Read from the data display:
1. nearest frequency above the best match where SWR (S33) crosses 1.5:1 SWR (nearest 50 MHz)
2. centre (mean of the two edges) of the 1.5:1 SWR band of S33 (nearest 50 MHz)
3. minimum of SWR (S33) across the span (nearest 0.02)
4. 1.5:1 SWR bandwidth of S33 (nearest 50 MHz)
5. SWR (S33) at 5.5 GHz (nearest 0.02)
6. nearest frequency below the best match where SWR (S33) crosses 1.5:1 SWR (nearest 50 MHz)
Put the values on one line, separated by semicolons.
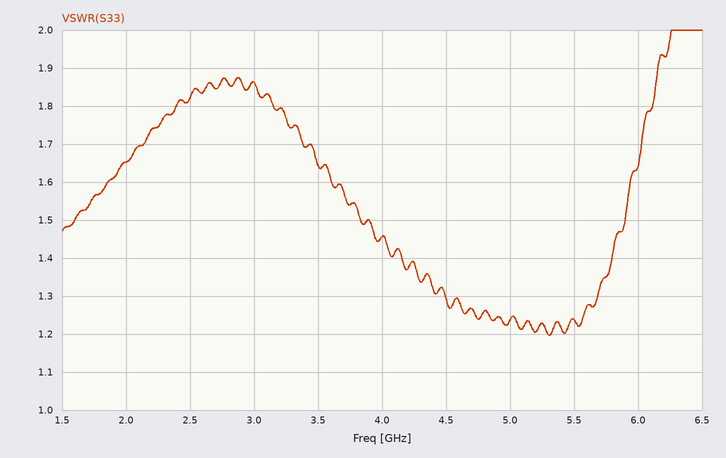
5.90 GHz; 4.90 GHz; 1.20; 2.00 GHz; 1.24; 3.90 GHz
